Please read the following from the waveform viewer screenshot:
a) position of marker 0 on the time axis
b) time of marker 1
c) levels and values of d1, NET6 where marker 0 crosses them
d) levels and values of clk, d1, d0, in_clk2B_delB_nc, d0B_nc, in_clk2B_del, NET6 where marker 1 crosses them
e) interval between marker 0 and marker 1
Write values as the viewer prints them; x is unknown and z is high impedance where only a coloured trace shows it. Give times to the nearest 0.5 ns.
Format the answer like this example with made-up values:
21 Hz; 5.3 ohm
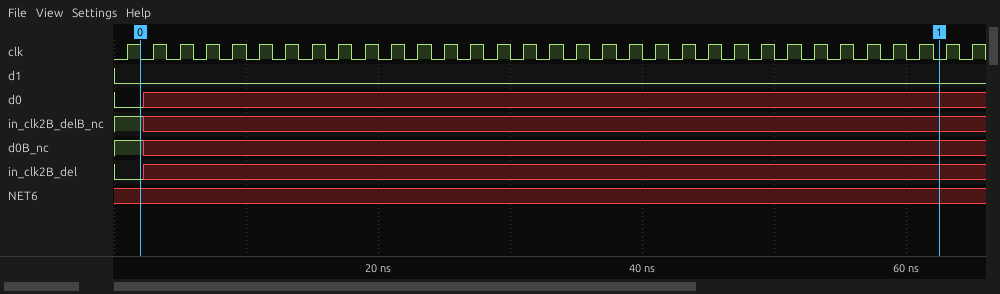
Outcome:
2 ns; 62.5 ns; d1=0, NET6=x; clk=0, d1=0, d0=x, in_clk2B_delB_nc=x, d0B_nc=x, in_clk2B_del=x, NET6=x; 60.5 ns
